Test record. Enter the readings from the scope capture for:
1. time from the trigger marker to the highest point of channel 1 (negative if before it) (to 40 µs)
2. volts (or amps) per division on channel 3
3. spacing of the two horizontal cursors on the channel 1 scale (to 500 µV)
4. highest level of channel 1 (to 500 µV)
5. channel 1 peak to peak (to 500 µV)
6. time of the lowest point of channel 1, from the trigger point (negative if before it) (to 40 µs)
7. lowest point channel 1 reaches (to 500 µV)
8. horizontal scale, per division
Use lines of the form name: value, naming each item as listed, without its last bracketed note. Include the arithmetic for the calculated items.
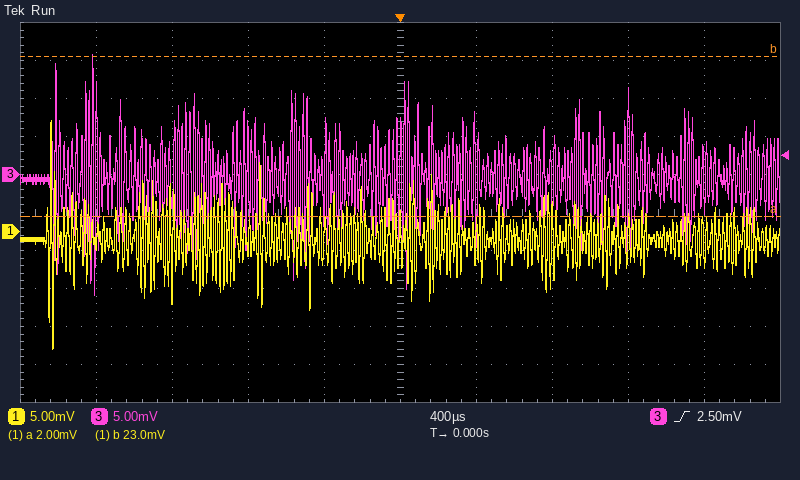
time from the trigger marker to the highest point of channel 1 (negative if before it): -1.84 ms
volts (or amps) per division on channel 3: 5 mV
spacing of the two horizontal cursors on the channel 1 scale: 21.0 mV
highest level of channel 1: 14.5 mV
channel 1 peak to peak: 14.5 mV − (-15.5 mV) = 30.0 mV
time of the lowest point of channel 1, from the trigger point (negative if before it): -1.84 ms
lowest point channel 1 reaches: -15.5 mV
horizontal scale, per division: 400 µs
